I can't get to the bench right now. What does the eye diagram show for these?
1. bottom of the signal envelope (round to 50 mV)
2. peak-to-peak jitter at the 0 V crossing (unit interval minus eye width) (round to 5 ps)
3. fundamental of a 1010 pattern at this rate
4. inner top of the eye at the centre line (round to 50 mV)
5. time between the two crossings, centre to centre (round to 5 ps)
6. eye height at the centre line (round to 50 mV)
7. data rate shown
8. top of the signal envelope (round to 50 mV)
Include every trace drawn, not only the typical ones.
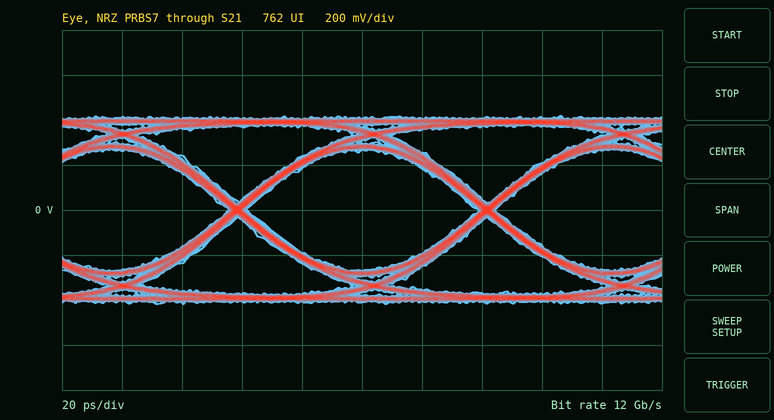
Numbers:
-400 mV
5 ps
6 GHz
250 mV
85 ps
550 mV
12 Gb/s
400 mV
